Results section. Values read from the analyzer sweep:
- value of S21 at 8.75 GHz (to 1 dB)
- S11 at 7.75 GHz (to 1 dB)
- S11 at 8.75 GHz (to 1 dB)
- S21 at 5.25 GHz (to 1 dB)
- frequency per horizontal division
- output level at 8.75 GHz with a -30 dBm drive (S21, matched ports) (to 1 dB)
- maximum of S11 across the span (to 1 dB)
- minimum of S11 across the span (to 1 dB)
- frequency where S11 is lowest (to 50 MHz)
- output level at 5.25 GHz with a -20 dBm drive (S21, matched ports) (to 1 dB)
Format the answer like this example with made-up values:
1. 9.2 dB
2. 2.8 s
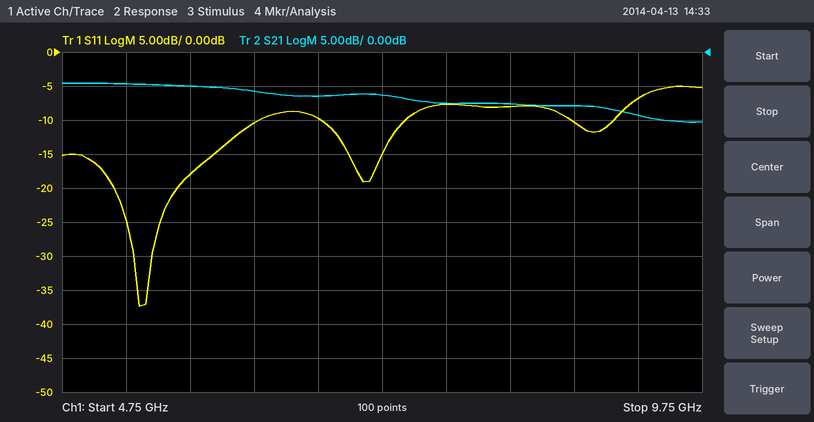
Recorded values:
1. -8 dB
2. -8 dB
3. -10 dB
4. -5 dB
5. 500 MHz
6. -38 dBm
7. -5 dB
8. -37 dB
9. 5.35 GHz
10. -25 dBm
